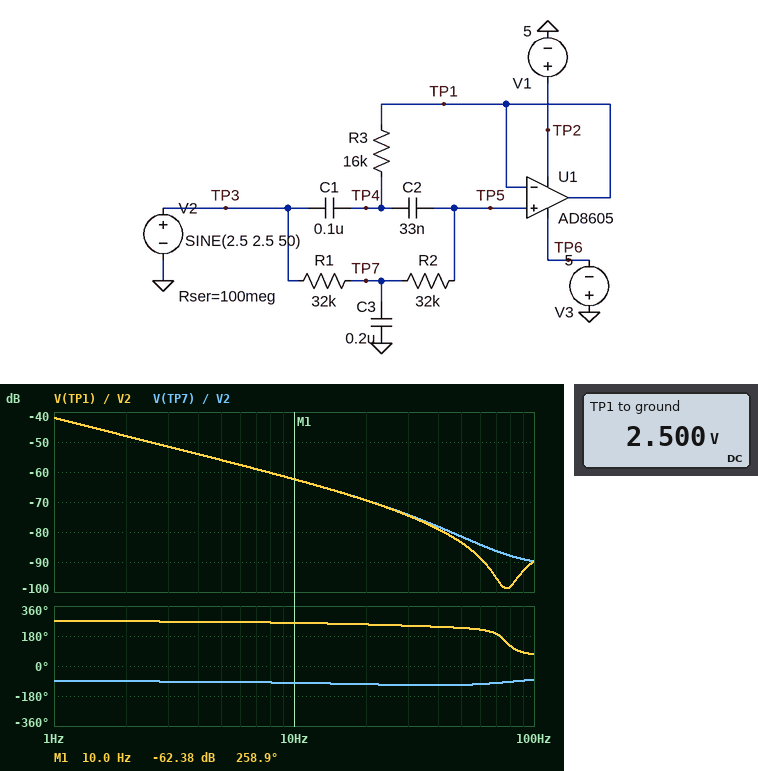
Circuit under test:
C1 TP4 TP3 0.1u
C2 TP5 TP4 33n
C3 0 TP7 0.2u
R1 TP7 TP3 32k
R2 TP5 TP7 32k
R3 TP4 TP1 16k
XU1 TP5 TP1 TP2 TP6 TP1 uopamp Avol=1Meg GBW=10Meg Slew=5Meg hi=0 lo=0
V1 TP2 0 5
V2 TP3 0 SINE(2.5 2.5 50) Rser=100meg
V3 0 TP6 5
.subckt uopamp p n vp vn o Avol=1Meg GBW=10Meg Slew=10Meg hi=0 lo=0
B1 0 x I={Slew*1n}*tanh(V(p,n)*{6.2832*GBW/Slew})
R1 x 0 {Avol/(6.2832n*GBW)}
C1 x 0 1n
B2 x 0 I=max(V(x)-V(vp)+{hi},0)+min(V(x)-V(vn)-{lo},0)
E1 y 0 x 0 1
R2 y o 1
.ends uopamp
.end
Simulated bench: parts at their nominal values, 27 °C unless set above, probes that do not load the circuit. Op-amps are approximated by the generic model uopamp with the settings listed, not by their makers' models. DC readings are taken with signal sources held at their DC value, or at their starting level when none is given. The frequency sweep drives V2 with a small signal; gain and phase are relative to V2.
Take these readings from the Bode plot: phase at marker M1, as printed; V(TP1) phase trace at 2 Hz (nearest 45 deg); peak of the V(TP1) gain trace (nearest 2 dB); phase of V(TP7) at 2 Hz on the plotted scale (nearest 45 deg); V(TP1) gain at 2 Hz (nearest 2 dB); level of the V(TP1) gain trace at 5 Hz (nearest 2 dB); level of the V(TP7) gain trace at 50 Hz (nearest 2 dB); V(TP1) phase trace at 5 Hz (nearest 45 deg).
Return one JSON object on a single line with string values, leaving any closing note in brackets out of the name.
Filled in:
{"phase at marker M1, as printed": "258.9 deg", "V(TP1) phase trace at 2 Hz": "270 deg", "peak of the V(TP1) gain trace": "-42 dB", "phase of V(TP7) at 2 Hz on the plotted scale": "-90 deg", "V(TP1) gain at 2 Hz": "-48 dB", "level of the V(TP1) gain trace at 5 Hz": "-56 dB", "level of the V(TP7) gain trace at 50 Hz": "-82 dB", "V(TP1) phase trace at 5 Hz": "270 deg"}
